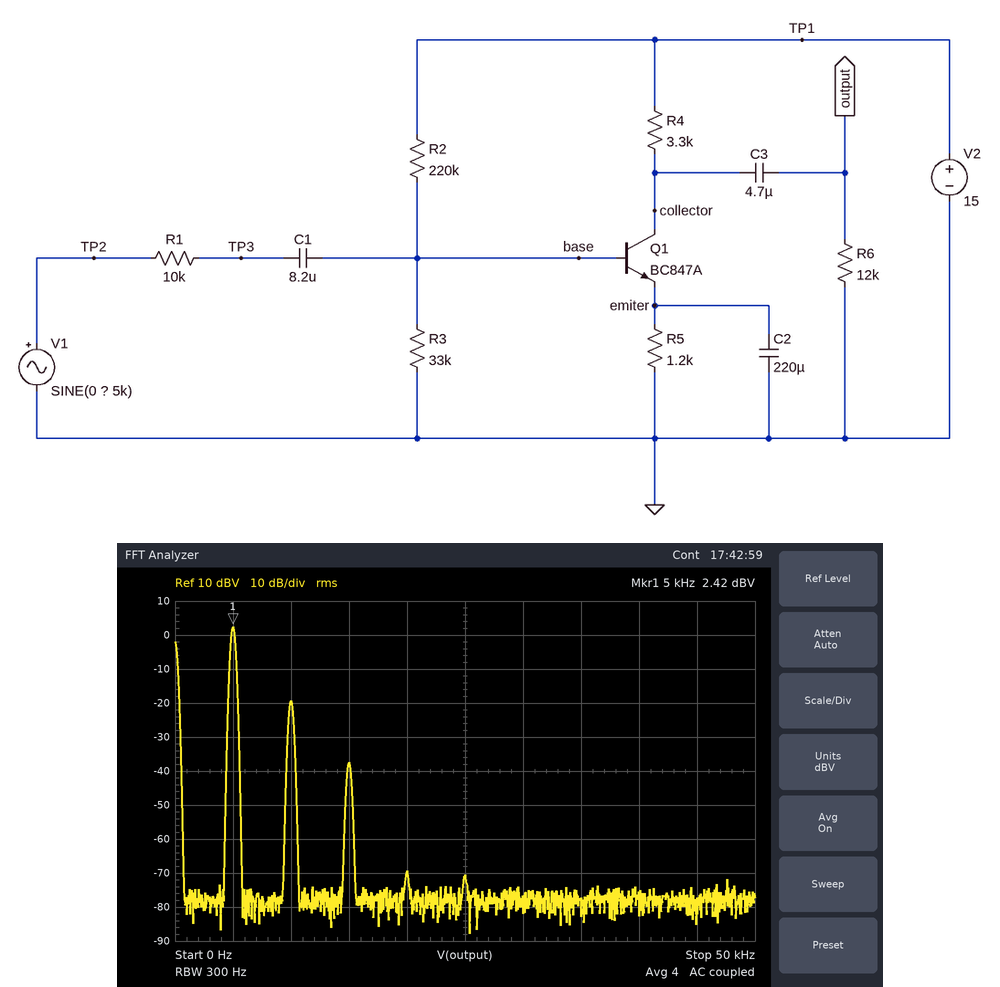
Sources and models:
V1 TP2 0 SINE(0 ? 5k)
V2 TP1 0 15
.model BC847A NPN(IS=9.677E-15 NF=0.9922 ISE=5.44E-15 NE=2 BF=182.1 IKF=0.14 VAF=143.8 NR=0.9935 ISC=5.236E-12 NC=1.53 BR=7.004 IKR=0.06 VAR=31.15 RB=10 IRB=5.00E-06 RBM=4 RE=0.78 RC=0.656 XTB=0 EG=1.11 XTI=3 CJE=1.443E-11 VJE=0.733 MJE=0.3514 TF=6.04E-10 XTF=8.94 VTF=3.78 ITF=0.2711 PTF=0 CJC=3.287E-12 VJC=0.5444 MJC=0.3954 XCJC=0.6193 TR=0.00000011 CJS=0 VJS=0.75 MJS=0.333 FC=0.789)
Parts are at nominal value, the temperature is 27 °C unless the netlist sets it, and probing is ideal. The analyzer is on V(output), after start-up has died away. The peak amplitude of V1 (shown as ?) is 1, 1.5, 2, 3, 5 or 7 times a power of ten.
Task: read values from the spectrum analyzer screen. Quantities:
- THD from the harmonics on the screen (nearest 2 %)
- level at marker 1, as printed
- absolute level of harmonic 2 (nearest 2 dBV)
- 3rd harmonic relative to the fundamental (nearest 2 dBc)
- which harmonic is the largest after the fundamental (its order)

8 %
2.42 dBV
-20 dBV
-40 dBc
2
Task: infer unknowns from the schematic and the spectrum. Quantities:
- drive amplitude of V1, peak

70 mV
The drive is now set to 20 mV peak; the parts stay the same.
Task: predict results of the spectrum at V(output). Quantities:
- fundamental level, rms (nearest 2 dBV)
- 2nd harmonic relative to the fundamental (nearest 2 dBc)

-8 dBV
-34 dBc
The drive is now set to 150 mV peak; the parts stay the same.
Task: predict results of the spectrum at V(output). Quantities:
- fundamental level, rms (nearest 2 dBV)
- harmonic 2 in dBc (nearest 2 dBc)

8 dBV
-12 dBc
